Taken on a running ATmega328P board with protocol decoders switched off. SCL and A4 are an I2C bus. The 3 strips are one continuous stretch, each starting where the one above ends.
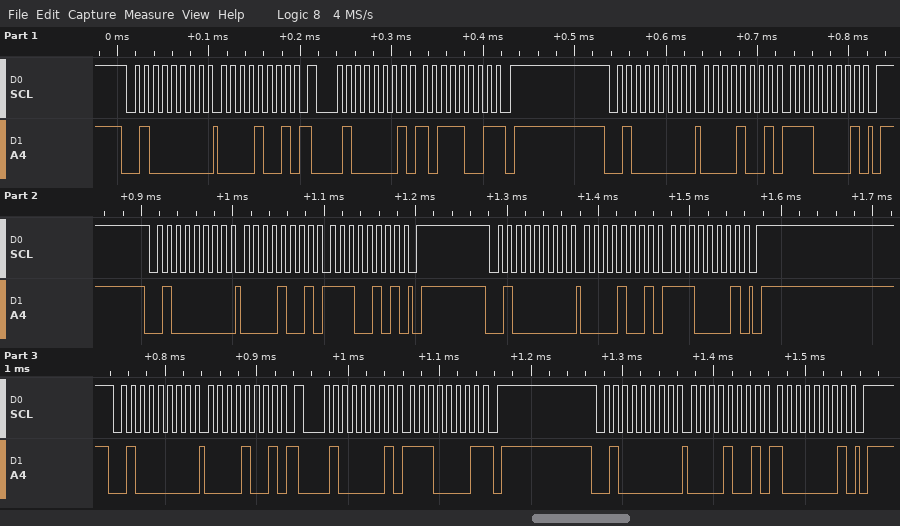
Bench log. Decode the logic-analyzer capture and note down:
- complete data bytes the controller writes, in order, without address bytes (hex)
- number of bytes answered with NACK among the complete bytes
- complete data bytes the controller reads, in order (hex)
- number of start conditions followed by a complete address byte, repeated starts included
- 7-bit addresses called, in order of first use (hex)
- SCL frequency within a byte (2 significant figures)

09 09 E1 09 E5 09 E1 09 09 81
2
B9 E1
8
0x20
100 kHz
